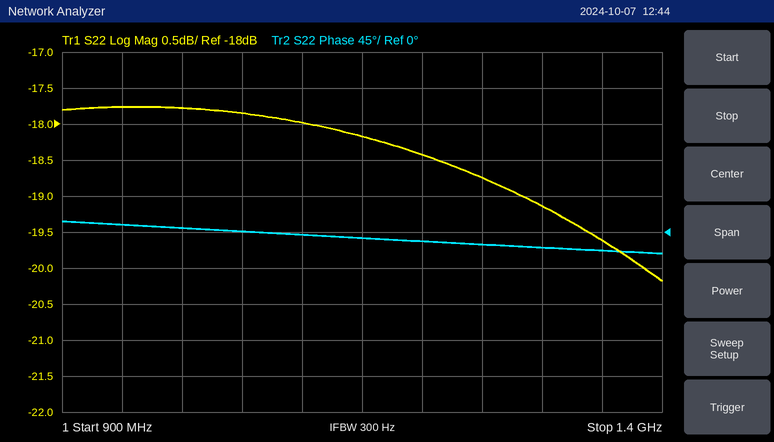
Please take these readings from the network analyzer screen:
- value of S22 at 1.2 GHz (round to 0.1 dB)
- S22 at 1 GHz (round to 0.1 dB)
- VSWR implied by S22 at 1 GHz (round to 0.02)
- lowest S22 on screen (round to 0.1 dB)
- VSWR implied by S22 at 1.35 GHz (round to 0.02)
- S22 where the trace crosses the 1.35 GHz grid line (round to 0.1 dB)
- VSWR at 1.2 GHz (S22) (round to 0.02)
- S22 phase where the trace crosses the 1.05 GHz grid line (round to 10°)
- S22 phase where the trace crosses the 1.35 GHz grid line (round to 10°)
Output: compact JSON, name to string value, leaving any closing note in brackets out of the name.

{"value of S22 at 1.2 GHz": "-18.4 dB", "S22 at 1 GHz": "-17.8 dB", "VSWR implied by S22 at 1 GHz": "1.30", "lowest S22 on screen": "-20.2 dB", "VSWR implied by S22 at 1.35 GHz": "1.24", "S22 where the trace crosses the 1.35 GHz grid line": "-19.6 dB", "VSWR at 1.2 GHz (S22)": "1.28", "S22 phase where the trace crosses the 1.05 GHz grid line": "0°", "S22 phase where the trace crosses the 1.35 GHz grid line": "-20°"}
